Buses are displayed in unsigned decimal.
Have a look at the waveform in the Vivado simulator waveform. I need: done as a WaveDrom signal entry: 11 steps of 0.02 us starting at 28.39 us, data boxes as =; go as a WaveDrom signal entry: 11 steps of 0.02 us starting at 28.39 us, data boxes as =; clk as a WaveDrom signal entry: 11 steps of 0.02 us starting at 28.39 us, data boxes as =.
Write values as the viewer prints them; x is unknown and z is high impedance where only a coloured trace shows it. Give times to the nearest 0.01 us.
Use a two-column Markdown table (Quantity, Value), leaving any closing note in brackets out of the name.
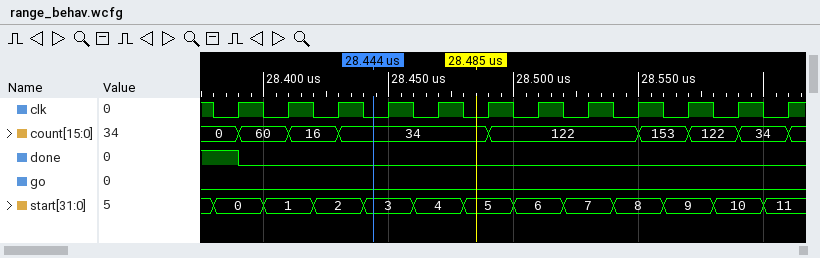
| Quantity | Value |
|---|---|
| done as a WaveDrom signal entry: 11 steps of 0.02 us starting at 28.39 us, data boxes as = | {name: 'done', wave: '0..........'} |
| go as a WaveDrom signal entry: 11 steps of 0.02 us starting at 28.39 us, data boxes as = | {name: 'go', wave: '0..........'} |
| clk as a WaveDrom signal entry: 11 steps of 0.02 us starting at 28.39 us, data boxes as = | {name: 'clk', wave: 'p..........'} |
